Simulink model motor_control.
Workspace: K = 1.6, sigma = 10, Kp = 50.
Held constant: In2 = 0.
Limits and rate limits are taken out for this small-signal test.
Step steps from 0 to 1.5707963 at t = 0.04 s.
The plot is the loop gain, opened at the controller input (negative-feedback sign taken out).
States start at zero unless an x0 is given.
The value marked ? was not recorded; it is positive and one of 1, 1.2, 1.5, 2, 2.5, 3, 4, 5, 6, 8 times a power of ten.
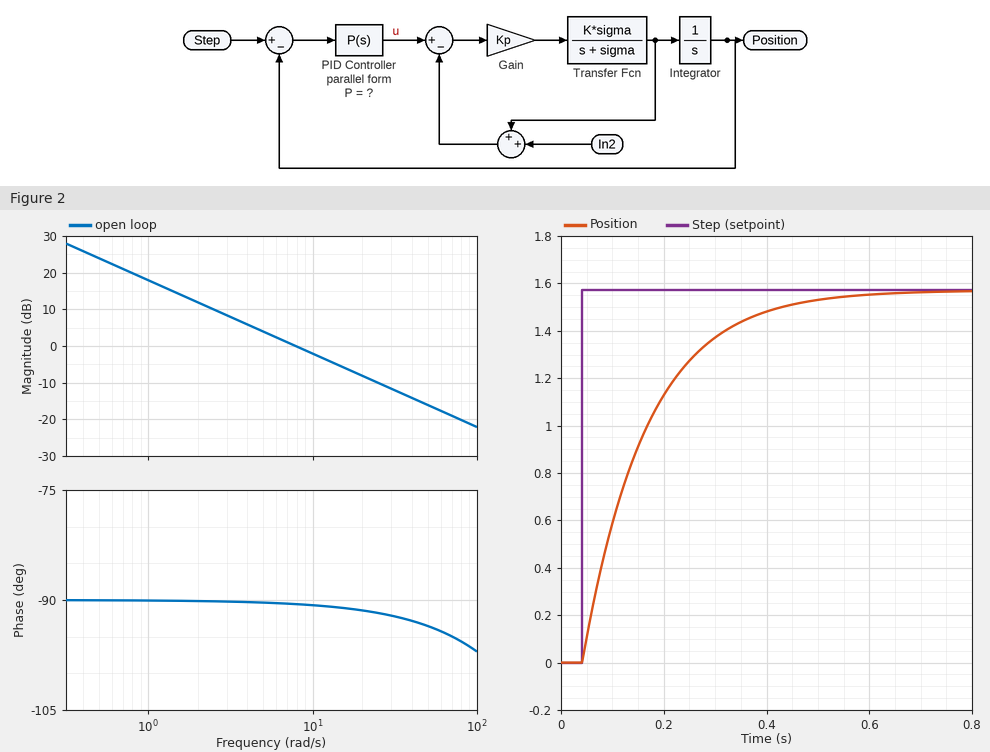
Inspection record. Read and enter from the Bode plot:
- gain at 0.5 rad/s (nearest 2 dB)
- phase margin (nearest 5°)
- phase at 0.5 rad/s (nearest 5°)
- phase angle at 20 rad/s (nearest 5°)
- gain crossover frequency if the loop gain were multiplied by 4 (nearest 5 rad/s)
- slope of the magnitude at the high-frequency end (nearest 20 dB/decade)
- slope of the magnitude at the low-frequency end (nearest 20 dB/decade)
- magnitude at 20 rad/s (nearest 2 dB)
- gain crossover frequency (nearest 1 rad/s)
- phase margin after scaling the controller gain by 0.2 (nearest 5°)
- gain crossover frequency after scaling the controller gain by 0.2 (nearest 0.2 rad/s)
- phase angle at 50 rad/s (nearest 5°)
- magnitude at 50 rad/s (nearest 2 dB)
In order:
24 dB
90°
-90°
-90°
30 rad/s
-20 dB/decade
-20 dB/decade
-8 dB
8 rad/s
90°
1.6 rad/s
-95°
-16 dB
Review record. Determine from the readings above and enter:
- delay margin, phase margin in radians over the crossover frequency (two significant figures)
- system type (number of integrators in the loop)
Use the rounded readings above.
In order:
0.20 s
1
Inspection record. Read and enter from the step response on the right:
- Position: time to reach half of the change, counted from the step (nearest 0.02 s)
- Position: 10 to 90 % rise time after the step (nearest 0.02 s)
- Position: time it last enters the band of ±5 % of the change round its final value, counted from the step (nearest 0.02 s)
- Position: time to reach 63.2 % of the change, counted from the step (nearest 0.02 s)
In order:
0.08 s
0.28 s
0.38 s
0.12 s
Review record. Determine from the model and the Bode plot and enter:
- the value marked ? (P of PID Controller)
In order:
8
